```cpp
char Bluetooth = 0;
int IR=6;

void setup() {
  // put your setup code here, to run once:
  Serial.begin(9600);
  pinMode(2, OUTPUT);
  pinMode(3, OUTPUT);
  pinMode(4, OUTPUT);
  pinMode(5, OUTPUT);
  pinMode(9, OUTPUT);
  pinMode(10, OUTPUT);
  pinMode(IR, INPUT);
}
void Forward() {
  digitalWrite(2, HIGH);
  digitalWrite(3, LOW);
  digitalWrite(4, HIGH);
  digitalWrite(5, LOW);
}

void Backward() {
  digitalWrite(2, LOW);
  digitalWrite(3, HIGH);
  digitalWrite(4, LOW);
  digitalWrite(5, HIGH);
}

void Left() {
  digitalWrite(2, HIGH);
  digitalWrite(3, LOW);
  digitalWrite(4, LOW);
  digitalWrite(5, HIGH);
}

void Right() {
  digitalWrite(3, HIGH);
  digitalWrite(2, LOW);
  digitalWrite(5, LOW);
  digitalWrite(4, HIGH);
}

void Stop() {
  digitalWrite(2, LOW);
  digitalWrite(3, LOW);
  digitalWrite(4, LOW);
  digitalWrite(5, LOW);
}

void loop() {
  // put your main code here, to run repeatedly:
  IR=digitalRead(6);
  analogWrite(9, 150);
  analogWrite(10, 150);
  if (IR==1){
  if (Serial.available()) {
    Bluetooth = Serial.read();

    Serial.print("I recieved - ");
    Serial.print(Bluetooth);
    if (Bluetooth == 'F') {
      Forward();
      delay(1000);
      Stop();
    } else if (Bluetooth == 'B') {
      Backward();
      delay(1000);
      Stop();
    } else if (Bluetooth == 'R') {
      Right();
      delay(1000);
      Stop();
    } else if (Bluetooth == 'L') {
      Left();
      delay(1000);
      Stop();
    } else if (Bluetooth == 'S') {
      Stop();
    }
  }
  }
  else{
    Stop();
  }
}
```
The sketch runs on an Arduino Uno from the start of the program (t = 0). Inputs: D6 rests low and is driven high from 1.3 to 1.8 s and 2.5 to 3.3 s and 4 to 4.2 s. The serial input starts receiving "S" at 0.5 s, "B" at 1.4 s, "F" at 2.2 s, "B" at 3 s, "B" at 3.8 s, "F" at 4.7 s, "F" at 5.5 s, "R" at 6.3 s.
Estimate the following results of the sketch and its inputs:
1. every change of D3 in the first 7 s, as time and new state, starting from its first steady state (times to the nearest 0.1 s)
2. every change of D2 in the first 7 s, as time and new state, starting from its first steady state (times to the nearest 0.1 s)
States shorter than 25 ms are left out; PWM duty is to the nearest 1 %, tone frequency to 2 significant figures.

0 s low; 1.4 s high; 2.4 s low; 4 s high; 5 s low
0 s low; 2.5 s high; 3.5 s low
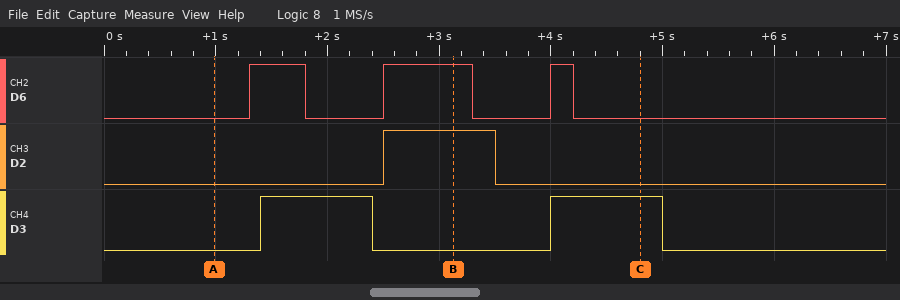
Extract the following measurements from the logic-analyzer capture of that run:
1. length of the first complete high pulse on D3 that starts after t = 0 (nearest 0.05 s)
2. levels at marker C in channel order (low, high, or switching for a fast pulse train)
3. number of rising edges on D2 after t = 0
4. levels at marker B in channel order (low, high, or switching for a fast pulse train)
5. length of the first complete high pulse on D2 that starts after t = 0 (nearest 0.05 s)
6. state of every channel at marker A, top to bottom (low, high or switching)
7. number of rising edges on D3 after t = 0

1.00 s
D6 low, D2 low, D3 high
1
D6 high, D2 high, D3 low
1.00 s
D6 low, D2 low, D3 low
2
